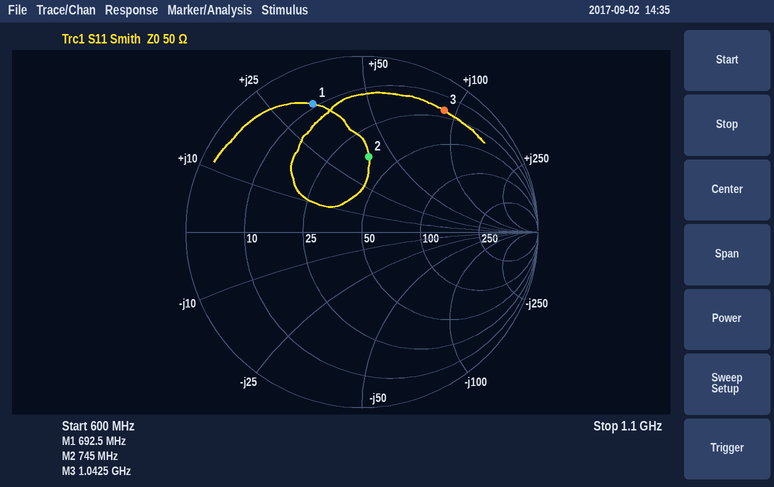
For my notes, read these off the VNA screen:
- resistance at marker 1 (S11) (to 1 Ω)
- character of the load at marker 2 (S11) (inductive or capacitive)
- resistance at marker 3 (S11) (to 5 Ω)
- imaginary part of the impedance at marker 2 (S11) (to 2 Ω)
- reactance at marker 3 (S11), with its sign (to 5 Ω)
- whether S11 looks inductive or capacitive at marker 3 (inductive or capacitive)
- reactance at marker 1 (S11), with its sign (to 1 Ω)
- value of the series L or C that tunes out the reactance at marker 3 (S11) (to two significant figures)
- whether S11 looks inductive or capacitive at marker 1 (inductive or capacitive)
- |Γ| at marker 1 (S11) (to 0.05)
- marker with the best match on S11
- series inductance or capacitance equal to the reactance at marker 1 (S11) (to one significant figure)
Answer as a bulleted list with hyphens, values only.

- 9 Ω
- inductive
- 20 Ω
- +38 Ω
- +90 Ω
- inductive
- +34 Ω
- 1.7 pF
- inductive
- 0.80
- marker 2
- 8 nH
